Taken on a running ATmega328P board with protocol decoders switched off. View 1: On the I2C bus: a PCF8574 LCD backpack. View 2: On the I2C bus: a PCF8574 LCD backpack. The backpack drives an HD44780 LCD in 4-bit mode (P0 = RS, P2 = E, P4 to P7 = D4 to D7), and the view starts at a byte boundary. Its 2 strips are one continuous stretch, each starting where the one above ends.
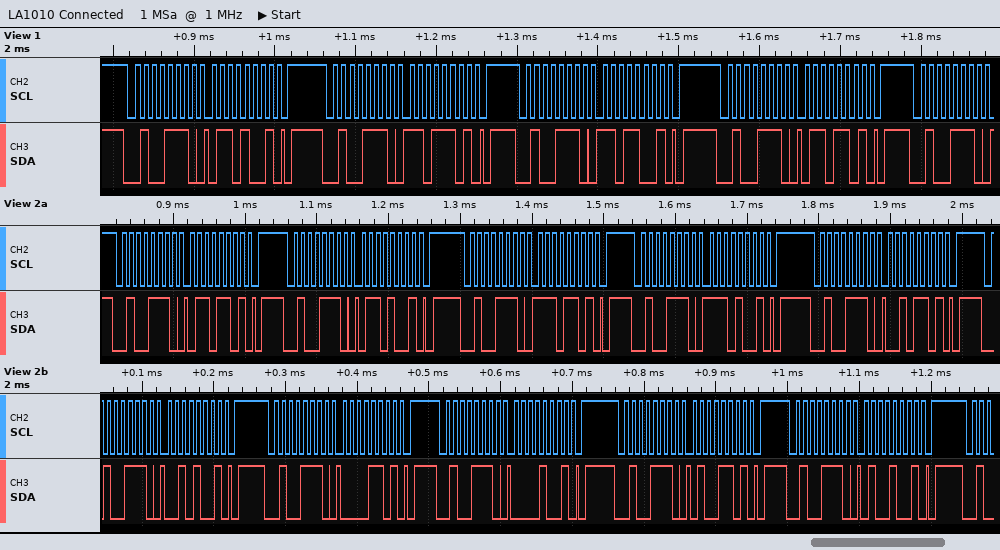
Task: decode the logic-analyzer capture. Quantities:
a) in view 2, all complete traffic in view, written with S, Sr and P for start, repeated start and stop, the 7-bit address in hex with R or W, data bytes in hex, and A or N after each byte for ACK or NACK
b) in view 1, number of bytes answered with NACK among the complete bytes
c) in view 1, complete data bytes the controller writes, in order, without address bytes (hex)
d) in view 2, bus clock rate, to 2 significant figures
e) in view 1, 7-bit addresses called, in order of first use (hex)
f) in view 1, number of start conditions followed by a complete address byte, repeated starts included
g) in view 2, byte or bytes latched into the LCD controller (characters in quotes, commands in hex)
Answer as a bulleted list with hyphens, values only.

- S 27W A 6D A P S 27W A 69 A P S 27W A ED A P S 27W A E9 A P S 27W A 2D A P S 27W A 29 A P S 27W A 0D A P S 27W A 09 A P S 27W A 4D A P S 27W A 49 A P
- 0
- 69 DD D9 6D
- 100 kHz
- 0x27
- 5
- 'n' ' '
